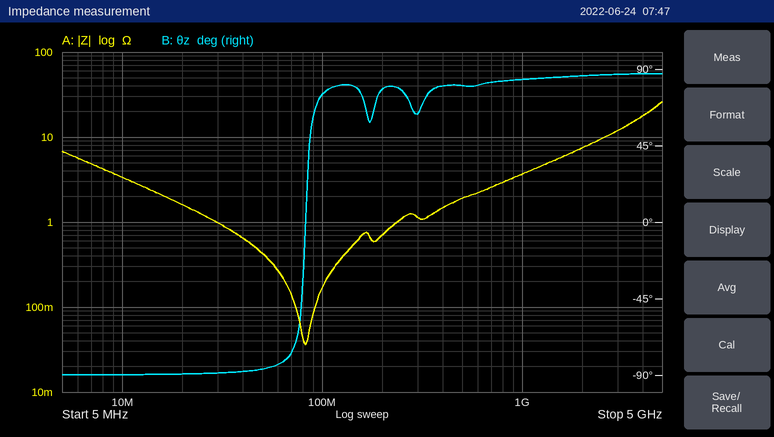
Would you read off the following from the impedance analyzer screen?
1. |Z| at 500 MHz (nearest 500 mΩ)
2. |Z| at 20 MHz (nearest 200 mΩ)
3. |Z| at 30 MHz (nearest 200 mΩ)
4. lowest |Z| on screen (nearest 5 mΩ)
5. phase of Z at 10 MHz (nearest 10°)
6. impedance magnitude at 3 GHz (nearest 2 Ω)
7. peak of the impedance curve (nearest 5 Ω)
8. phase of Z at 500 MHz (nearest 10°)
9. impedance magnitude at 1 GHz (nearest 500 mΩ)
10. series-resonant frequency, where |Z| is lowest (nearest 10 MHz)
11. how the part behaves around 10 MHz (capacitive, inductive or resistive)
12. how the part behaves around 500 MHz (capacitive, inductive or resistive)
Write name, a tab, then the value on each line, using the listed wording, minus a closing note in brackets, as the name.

|Z| at 500 MHz	2.0 Ω
|Z| at 20 MHz	1.6 Ω
|Z| at 30 MHz	1.0 Ω
lowest |Z| on screen	35 mΩ
phase of Z at 10 MHz	-90°
impedance magnitude at 3 GHz	12 Ω
peak of the impedance curve	25 Ω
phase of Z at 500 MHz	80°
impedance magnitude at 1 GHz	3.5 Ω
series-resonant frequency, where |Z| is lowest	80 MHz
how the part behaves around 10 MHz	capacitive
how the part behaves around 500 MHz	inductive
